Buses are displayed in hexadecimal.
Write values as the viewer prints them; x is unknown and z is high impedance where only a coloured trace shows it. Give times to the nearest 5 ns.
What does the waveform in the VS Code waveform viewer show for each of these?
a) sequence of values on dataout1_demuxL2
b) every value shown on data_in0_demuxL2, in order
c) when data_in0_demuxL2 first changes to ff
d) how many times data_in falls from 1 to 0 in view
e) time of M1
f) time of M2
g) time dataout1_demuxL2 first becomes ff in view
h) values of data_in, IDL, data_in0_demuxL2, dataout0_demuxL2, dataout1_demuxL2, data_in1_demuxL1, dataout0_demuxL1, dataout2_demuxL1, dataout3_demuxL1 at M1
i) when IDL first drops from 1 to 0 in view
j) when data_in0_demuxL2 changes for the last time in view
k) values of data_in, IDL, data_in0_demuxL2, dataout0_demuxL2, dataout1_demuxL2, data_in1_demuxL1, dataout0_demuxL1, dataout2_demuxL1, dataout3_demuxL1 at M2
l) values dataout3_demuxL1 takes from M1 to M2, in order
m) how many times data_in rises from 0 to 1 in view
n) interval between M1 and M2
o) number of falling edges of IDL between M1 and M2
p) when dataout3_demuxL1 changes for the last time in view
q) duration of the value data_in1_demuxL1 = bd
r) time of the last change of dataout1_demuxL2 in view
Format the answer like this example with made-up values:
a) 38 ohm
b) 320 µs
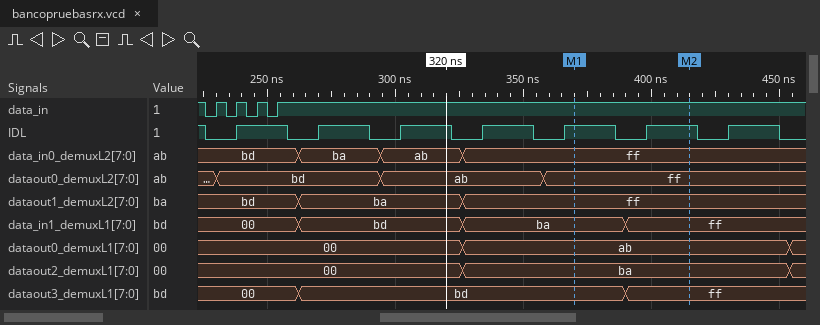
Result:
a) bd, ba, ff
b) bd, ba, ab, ff
c) 325 ns
d) 4
e) 370 ns
f) 415 ns
g) 325 ns
h) data_in=1, IDL=1, data_in0_demuxL2=ff, dataout0_demuxL2=ff, dataout1_demuxL2=ff, data_in1_demuxL1=ba, dataout0_demuxL1=ab, dataout2_demuxL1=ba, dataout3_demuxL1=bd
i) 225 ns
j) 325 ns
k) data_in=1, IDL=1, data_in0_demuxL2=ff, dataout0_demuxL2=ff, dataout1_demuxL2=ff, data_in1_demuxL1=ff, dataout0_demuxL1=ab, dataout2_demuxL1=ba, dataout3_demuxL1=ff
l) bd, ff
m) 4
n) 45 ns
o) 1
p) 390 ns
q) 65 ns
r) 325 ns
